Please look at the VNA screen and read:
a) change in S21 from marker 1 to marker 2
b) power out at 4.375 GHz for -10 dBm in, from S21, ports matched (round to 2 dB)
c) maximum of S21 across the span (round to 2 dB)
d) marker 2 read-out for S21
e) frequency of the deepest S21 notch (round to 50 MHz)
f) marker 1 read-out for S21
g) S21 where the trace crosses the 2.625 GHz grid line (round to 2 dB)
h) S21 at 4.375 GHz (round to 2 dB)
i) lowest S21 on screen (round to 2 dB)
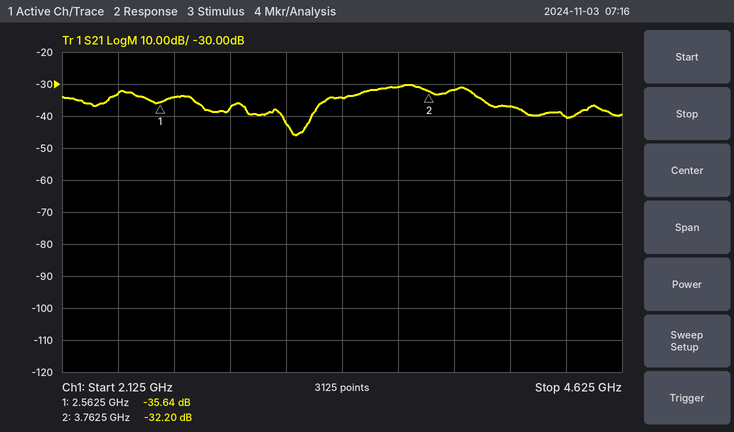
3.44 dB
-50 dBm
-30 dB
-32.20 dB
3.15 GHz
-35.64 dB
-34 dB
-40 dB
-46 dB
